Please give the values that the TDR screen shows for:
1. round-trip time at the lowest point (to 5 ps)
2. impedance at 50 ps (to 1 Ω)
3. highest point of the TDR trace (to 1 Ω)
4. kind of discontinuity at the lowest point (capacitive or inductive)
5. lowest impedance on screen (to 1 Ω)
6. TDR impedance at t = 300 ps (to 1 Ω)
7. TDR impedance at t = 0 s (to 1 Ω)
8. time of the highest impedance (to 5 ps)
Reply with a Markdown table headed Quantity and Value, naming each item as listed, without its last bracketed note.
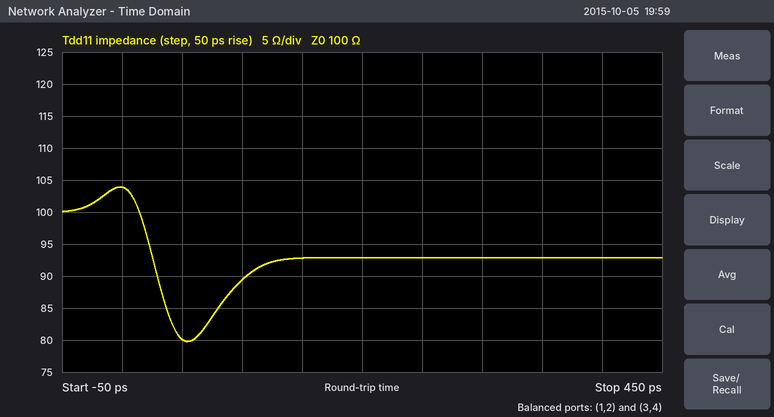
| Quantity | Value |
|---|---|
| round-trip time at the lowest point | 55 ps |
| impedance at 50 ps | 80 Ω |
| highest point of the TDR trace | 104 Ω |
| kind of discontinuity at the lowest point | capacitive |
| lowest impedance on screen | 80 Ω |
| TDR impedance at t = 300 ps | 93 Ω |
| TDR impedance at t = 0 s | 104 Ω |
| time of the highest impedance | 0 ps |
